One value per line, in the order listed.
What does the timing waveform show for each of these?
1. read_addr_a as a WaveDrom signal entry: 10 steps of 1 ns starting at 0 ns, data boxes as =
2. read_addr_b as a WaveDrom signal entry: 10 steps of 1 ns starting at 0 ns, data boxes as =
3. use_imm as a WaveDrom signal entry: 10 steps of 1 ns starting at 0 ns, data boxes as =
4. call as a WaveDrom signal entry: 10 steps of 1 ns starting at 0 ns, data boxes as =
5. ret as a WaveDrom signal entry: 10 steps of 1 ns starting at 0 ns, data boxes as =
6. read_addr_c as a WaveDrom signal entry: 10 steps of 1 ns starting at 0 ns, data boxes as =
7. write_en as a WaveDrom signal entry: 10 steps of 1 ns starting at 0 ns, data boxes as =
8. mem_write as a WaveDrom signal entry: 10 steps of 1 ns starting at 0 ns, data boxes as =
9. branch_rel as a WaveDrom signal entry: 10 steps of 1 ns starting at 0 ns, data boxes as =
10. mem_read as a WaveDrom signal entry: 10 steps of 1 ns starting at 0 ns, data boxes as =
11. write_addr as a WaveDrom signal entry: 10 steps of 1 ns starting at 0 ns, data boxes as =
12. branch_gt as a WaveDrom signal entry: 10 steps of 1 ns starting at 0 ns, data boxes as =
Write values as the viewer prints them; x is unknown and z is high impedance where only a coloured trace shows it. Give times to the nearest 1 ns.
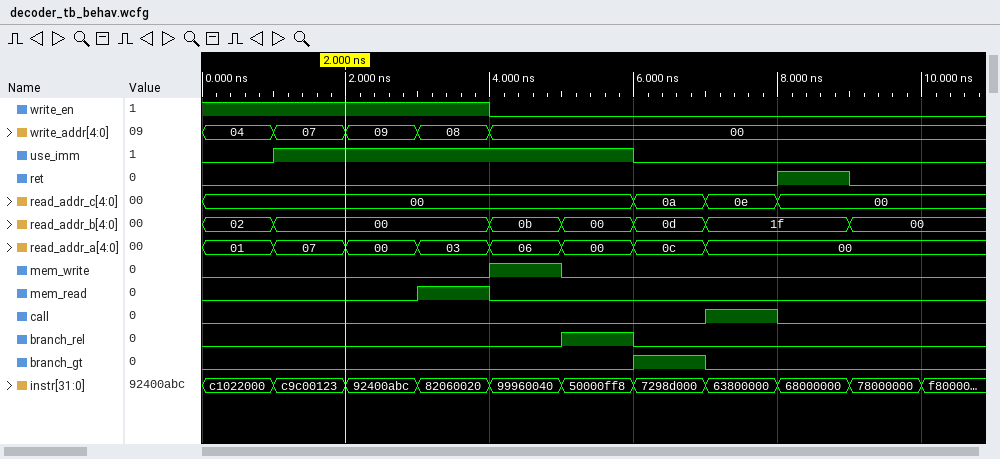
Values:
{name: 'read_addr_a', wave: '========..', data: '01 07 00 03 06 00 0c 00'}
{name: 'read_addr_b', wave: '==..====.=', data: '02 00 0b 00 0d 1f 00'}
{name: 'use_imm', wave: '01....0...'}
{name: 'call', wave: '0......10.'}
{name: 'ret', wave: '0.......10'}
{name: 'read_addr_c', wave: '=.....===.', data: '00 0a 0e 00'}
{name: 'write_en', wave: '1...0.....'}
{name: 'mem_write', wave: '0...10....'}
{name: 'branch_rel', wave: '0....10...'}
{name: 'mem_read', wave: '0..10.....'}
{name: 'write_addr', wave: '=====.....', data: '04 07 09 08 00'}
{name: 'branch_gt', wave: '0.....10..'}
